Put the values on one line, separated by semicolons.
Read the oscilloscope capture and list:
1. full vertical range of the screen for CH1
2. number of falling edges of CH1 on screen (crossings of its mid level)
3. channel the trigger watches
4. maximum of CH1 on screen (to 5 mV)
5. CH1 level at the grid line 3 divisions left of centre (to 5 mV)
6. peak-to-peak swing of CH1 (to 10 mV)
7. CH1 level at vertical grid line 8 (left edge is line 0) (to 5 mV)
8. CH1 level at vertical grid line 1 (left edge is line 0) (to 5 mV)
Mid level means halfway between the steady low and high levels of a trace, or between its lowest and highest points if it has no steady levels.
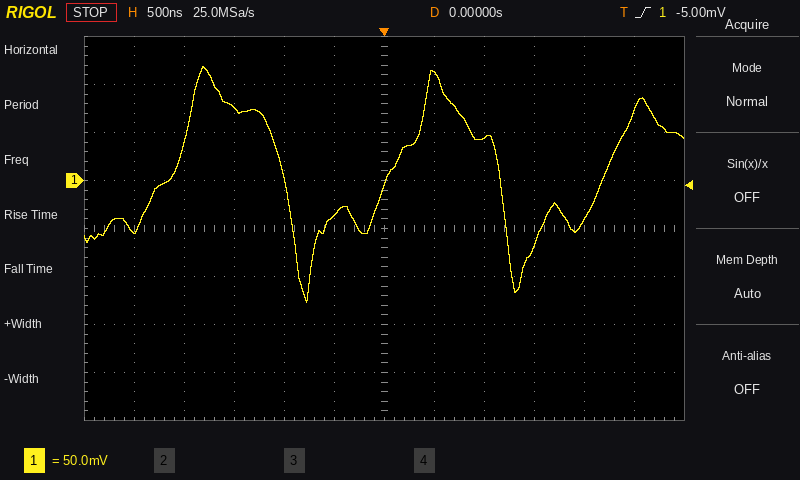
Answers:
400 mV; 2; CH1; 120 mV; 75 mV; 250 mV; 45 mV; -55 mV
